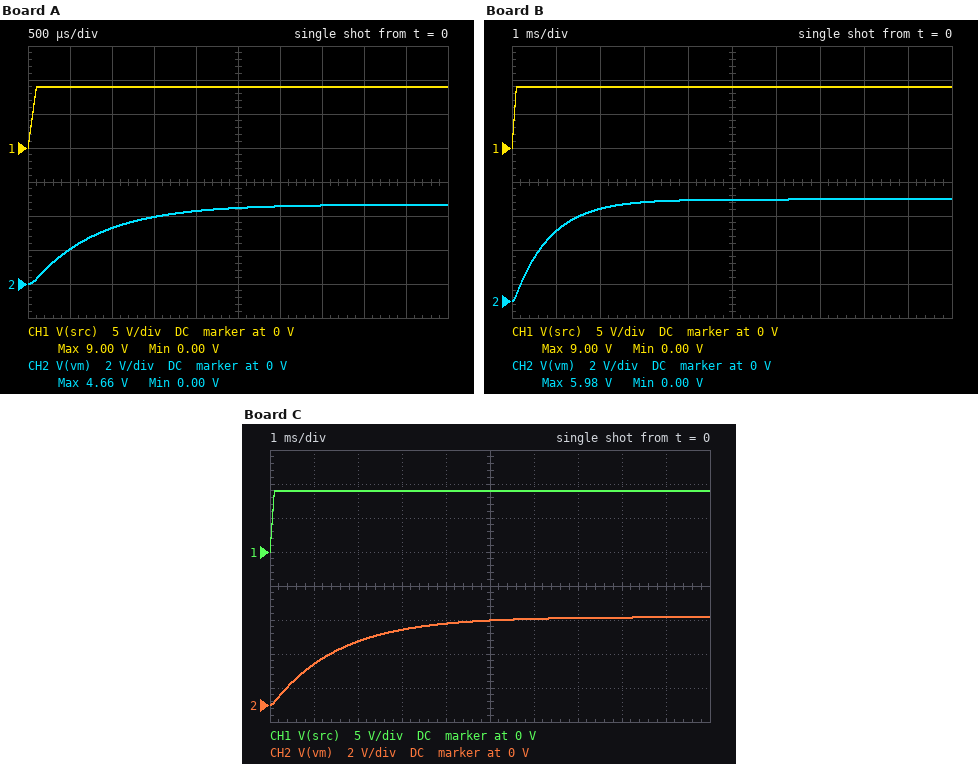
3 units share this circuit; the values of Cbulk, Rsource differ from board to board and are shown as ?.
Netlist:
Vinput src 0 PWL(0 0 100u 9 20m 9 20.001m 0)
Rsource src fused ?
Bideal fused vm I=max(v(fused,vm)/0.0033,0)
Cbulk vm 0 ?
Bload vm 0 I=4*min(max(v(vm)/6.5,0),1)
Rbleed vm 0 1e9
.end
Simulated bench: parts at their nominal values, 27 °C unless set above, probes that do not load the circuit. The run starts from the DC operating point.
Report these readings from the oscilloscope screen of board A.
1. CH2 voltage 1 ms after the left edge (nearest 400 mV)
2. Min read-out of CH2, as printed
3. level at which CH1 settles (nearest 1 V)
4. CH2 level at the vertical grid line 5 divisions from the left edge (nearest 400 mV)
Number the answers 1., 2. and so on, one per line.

1. 3.2 V
2. 0.00 V
3. 9 V
4. 4.4 V
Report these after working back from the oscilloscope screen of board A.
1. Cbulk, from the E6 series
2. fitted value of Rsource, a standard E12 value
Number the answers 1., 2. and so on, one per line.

1. 1 mF
2. 1.5 Ω
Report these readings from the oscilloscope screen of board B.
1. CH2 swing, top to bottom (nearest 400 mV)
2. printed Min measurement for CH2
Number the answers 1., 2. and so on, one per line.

1. 6.0 V
2. 0.00 V
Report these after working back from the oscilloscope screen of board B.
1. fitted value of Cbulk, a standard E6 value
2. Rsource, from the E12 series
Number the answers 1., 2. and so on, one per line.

1. 1.5 mF
2. 0.82 Ω
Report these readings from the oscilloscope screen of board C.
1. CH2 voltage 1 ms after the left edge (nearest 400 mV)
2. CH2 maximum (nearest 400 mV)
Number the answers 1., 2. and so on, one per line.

1. 2.4 V
2. 5.2 V
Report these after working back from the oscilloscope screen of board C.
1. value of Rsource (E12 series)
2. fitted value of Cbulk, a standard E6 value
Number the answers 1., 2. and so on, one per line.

1. 1.2 Ω
2. 2.2 mF
